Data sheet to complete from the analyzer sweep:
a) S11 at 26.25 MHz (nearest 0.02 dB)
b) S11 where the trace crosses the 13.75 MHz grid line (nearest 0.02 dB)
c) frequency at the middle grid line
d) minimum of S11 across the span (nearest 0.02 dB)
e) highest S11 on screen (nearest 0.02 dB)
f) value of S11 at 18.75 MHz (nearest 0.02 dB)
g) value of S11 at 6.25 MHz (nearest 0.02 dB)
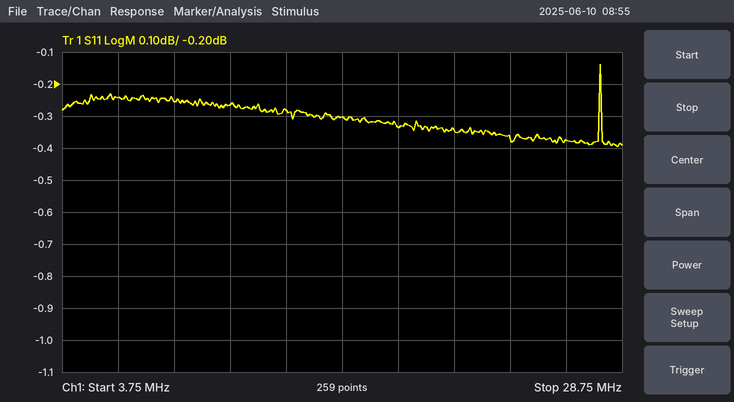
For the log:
-0.38 dB
-0.28 dB
16.25 MHz
-0.40 dB
-0.14 dB
-0.34 dB
-0.24 dB
